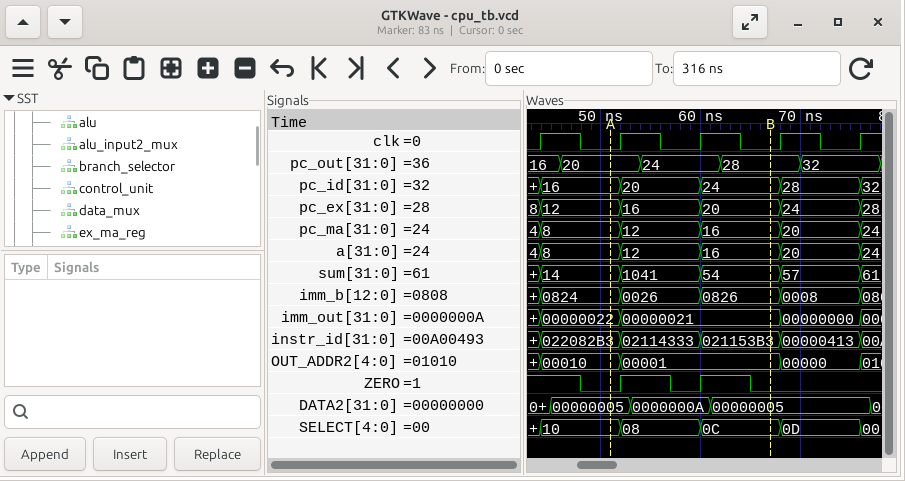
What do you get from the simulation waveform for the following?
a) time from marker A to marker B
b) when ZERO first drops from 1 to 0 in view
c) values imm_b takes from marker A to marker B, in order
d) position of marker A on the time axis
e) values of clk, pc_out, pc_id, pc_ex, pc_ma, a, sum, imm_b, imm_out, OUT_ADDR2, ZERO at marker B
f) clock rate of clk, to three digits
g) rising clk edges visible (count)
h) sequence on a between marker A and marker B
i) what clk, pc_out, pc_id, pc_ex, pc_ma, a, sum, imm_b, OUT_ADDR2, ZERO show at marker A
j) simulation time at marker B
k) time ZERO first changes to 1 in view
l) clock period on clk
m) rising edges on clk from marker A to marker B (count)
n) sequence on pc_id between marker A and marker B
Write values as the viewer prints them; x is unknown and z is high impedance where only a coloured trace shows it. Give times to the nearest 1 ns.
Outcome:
16 ns
48 ns
0824, 0026, 0826
51 ns
clk=0, pc_out=28, pc_id=24, pc_ex=20, pc_ma=16, a=16, sum=54, imm_b=0826, imm_out=00000021, OUT_ADDR2=00001, ZERO=0
125 MHz
5
8, 12, 16
clk=0, pc_out=20, pc_id=16, pc_ex=12, pc_ma=8, a=8, sum=14, imm_b=0824, OUT_ADDR2=00010, ZERO=0
67 ns
52 ns
8 ns
2
16, 20, 24
